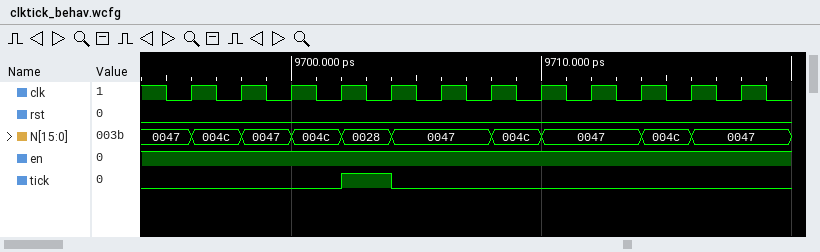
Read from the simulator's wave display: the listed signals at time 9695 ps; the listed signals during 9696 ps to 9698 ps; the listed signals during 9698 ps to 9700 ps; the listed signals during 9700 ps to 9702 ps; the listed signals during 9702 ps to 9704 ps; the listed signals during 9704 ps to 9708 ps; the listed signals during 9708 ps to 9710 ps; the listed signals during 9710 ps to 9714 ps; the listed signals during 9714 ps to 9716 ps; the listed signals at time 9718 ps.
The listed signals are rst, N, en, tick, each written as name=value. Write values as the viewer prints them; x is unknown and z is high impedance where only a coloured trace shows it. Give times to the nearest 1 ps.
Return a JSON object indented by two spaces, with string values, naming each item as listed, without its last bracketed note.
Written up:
{
  "the listed signals at time 9695 ps": "rst=0, N=0047, en=1, tick=0",
  "the listed signals during 9696 ps to 9698 ps": "rst=0, N=004c, en=1, tick=0",
  "the listed signals during 9698 ps to 9700 ps": "rst=0, N=0047, en=1, tick=0",
  "the listed signals during 9700 ps to 9702 ps": "rst=0, N=004c, en=1, tick=0",
  "the listed signals during 9702 ps to 9704 ps": "rst=0, N=0028, en=1, tick=1",
  "the listed signals during 9704 ps to 9708 ps": "rst=0, N=0047, en=1, tick=0",
  "the listed signals during 9708 ps to 9710 ps": "rst=0, N=004c, en=1, tick=0",
  "the listed signals during 9710 ps to 9714 ps": "rst=0, N=0047, en=1, tick=0",
  "the listed signals during 9714 ps to 9716 ps": "rst=0, N=004c, en=1, tick=0",
  "the listed signals at time 9718 ps": "rst=0, N=0047, en=1, tick=0"
}
